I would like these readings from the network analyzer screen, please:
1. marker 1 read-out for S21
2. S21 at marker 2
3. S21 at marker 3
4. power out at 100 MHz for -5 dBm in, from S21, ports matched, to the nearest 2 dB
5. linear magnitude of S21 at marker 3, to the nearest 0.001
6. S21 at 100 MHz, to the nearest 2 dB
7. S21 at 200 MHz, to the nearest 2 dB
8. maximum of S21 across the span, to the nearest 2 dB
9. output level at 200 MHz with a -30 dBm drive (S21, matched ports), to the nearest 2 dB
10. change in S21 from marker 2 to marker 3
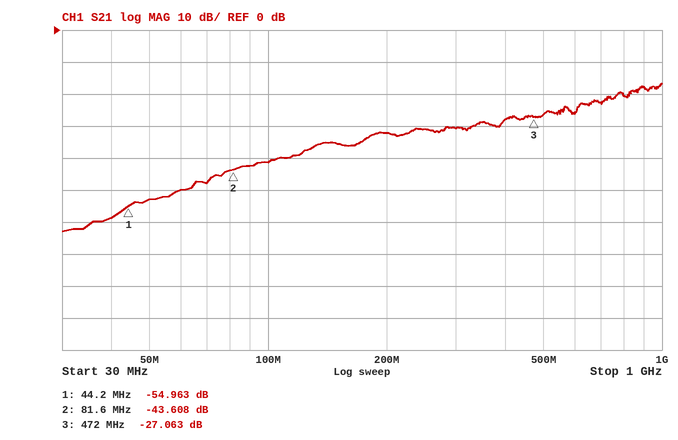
-54.963 dB
-43.608 dB
-27.063 dB
-46 dBm
0.044
-42 dB
-32 dB
-16 dB
-62 dBm
16.545 dB
